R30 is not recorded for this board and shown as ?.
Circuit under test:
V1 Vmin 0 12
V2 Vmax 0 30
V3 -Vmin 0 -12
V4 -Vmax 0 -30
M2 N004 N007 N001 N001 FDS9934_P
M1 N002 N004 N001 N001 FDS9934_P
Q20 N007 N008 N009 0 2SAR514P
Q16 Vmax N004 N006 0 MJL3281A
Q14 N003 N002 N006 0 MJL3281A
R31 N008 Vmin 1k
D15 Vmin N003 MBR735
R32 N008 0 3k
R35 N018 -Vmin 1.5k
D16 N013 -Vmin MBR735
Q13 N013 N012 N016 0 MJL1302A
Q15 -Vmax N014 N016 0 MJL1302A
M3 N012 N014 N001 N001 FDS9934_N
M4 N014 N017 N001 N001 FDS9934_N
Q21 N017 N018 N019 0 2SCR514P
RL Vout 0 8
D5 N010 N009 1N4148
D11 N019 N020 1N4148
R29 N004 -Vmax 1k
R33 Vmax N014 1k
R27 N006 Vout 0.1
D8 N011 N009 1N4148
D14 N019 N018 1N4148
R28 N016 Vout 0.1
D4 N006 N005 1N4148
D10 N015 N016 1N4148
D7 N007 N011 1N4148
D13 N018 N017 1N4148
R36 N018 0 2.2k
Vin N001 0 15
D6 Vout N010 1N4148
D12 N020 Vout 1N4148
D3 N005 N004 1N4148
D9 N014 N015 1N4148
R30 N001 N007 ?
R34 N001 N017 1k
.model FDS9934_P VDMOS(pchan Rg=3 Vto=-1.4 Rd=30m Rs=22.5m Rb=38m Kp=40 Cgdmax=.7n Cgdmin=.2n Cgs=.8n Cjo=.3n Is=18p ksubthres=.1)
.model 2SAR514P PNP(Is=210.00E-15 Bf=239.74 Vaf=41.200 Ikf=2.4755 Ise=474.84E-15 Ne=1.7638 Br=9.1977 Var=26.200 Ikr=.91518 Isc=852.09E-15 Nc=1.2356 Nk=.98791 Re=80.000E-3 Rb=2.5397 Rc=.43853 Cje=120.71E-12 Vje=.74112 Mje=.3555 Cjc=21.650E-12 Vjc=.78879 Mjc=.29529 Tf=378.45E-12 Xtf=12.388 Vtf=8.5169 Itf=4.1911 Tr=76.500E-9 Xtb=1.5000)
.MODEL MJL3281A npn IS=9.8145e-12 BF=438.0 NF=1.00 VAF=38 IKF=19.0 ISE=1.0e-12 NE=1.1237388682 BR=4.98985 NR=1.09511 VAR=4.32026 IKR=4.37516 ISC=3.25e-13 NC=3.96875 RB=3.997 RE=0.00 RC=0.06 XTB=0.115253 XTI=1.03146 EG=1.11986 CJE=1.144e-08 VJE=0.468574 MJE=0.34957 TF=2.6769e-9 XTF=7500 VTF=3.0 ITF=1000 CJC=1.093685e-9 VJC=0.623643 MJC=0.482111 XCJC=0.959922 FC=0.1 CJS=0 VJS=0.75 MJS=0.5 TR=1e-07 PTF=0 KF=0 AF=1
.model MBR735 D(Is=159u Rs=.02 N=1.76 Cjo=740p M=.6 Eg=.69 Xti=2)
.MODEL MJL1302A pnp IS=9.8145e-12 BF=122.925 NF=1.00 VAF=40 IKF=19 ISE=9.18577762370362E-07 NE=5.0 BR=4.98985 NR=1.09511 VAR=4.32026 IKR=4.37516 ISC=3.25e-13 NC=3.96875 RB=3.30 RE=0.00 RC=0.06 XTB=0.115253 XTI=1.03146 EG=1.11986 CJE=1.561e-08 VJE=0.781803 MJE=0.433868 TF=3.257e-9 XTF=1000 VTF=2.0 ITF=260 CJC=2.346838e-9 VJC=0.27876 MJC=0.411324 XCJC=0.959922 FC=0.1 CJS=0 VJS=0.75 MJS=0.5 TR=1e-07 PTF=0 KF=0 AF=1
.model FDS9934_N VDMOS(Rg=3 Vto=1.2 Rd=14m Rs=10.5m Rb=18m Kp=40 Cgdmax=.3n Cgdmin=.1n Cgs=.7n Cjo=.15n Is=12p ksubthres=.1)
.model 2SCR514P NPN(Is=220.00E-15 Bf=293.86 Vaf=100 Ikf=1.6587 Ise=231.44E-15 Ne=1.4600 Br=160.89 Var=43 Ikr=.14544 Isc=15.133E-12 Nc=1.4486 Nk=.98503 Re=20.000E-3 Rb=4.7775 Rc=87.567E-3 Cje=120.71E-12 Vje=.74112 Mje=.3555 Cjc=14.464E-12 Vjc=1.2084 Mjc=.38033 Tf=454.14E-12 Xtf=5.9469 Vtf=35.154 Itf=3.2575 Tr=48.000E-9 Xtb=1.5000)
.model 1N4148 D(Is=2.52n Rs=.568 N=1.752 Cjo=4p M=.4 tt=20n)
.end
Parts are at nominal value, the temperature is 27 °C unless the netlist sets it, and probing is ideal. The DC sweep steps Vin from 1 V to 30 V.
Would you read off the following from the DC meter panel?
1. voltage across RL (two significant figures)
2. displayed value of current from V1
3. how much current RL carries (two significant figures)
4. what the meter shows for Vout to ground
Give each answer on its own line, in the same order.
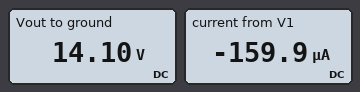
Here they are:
14 V
-159.9 µA
1.8 A
14.10 V
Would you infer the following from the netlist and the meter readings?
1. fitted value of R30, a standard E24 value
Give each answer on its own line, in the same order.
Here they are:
1.6 kΩ
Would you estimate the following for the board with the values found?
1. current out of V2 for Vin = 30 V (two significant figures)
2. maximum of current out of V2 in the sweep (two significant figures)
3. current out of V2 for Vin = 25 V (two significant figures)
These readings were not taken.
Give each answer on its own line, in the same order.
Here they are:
3.6 A
3.6 A
3.0 A
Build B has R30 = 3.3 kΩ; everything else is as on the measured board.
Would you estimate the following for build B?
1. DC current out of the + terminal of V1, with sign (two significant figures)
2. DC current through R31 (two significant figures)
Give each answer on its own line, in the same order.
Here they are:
-140 µA
140 µA
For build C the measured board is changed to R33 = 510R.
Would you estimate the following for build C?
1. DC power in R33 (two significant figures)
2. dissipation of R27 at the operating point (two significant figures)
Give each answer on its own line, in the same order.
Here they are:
410 mW
300 mW
